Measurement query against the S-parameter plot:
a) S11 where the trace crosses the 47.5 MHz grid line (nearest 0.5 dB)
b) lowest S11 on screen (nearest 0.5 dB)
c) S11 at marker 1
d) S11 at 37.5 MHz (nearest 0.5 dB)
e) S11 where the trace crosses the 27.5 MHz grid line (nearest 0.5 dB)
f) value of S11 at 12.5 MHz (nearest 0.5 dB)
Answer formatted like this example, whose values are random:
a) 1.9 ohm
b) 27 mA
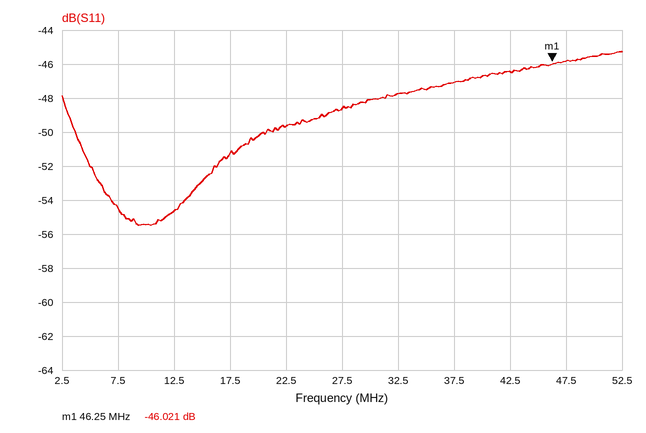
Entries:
a) -46.0 dB
b) -55.5 dB
c) -46.021 dB
d) -47.0 dB
e) -48.5 dB
f) -54.5 dB
